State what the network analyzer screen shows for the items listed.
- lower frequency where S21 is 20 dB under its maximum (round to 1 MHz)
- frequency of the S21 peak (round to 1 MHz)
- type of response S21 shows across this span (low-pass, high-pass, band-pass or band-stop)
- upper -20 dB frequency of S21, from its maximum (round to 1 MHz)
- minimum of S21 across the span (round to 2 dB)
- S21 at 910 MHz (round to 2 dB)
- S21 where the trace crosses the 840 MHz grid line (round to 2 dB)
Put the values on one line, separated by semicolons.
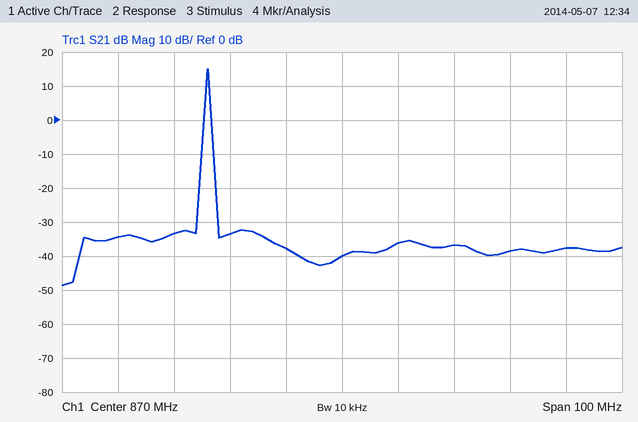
845 MHz; 846 MHz; band-pass; 847 MHz; -48 dB; -38 dB; -34 dB
